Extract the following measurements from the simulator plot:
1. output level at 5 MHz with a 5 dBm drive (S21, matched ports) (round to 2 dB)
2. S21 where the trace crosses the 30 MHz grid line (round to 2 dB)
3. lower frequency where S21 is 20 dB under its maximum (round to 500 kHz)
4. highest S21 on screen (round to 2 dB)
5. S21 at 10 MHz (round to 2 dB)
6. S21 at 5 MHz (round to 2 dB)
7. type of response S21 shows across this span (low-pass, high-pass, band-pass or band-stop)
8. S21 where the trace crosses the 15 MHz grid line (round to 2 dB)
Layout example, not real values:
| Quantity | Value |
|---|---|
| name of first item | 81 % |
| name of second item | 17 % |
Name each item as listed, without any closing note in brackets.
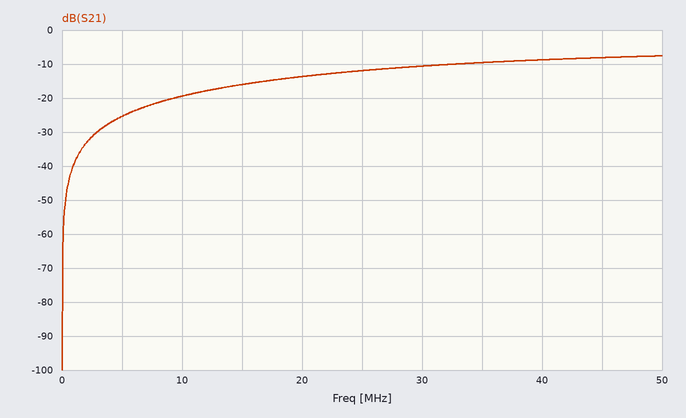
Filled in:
| Quantity | Value |
|---|---|
| output level at 5 MHz with a 5 dBm drive (S21, matched ports) | -20 dBm |
| S21 where the trace crosses the 30 MHz grid line | -10 dB |
| lower frequency where S21 is 20 dB under its maximum | 4.0 MHz |
| highest S21 on screen | -8 dB |
| S21 at 10 MHz | -20 dB |
| S21 at 5 MHz | -26 dB |
| type of response S21 shows across this span | high-pass |
| S21 where the trace crosses the 15 MHz grid line | -16 dB |
